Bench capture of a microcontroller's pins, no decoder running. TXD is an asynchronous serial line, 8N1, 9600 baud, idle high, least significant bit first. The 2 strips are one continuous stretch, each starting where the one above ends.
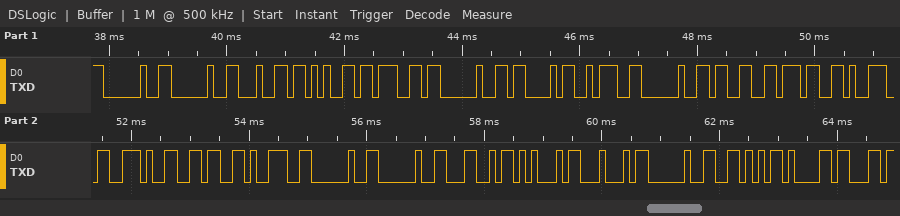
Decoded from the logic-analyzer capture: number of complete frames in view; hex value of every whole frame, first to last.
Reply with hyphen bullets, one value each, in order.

- 23
- 0x20 0x20 0x64 0x65 0x67 0x20 0x43 0x3A 0x20 0x33 0x37 0x39 0x2E 0x36 0x39 0x20 0x20 0x4C 0x45 0x44 0x20 0x56 0x61
